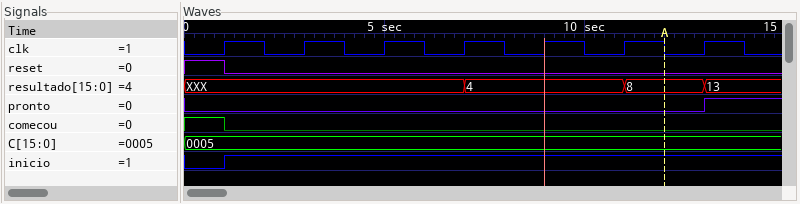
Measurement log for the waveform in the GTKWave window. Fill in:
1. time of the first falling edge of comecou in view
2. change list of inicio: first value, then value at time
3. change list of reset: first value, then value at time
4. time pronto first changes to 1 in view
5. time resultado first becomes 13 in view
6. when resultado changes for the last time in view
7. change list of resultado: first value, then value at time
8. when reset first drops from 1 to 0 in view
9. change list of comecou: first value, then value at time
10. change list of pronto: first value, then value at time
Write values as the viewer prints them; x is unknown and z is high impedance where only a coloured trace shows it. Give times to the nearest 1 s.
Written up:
1 s
0, 1 at 1 s
1, 0 at 1 s
13 s
13 s
13 s
XXX, 4 at 7 s, 8 at 11 s, 13 at 13 s
1 s
1, 0 at 1 s
0, 1 at 13 s
